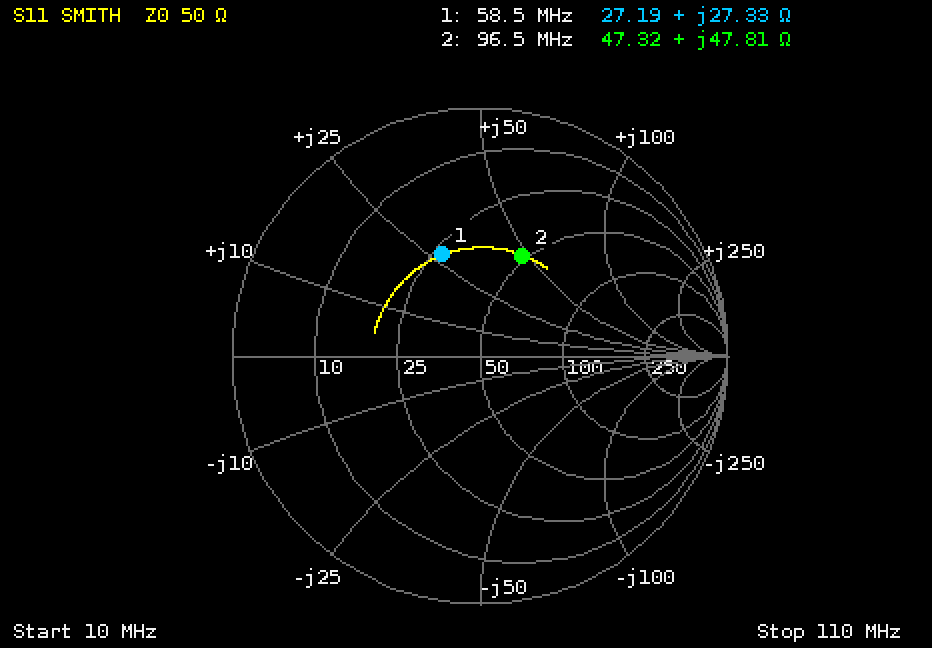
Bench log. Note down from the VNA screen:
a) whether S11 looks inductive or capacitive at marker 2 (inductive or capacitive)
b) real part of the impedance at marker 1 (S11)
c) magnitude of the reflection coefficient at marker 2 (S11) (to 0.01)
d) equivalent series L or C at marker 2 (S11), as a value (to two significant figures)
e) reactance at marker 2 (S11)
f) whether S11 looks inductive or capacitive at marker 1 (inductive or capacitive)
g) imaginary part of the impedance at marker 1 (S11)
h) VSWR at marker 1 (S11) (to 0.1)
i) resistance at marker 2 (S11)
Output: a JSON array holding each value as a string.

["inductive", "27.19 Ω", "0.44", "79 nH", "+47.81 Ω", "inductive", "+27.33 Ω", "2.5", "47.32 Ω"]
